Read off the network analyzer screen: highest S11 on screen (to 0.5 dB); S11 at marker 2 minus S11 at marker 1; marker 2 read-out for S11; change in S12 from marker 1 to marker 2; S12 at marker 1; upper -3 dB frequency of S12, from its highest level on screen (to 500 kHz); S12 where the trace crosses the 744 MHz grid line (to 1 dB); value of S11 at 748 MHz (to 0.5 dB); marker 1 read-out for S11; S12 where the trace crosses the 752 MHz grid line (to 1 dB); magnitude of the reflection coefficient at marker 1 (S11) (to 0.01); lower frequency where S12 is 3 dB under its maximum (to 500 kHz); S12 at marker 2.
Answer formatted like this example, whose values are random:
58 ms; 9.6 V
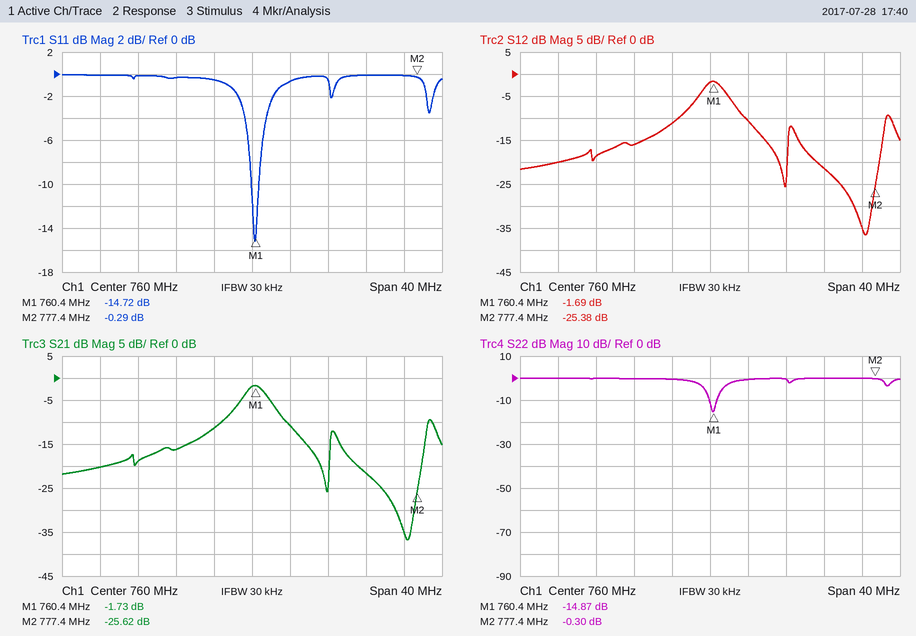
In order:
0.0 dB; 14.43 dB; -0.29 dB; -23.69 dB; -1.69 dB; 762.0 MHz; -20 dB; 0.0 dB; -14.72 dB; -16 dB; 0.18; 759.0 MHz; -25.38 dB
